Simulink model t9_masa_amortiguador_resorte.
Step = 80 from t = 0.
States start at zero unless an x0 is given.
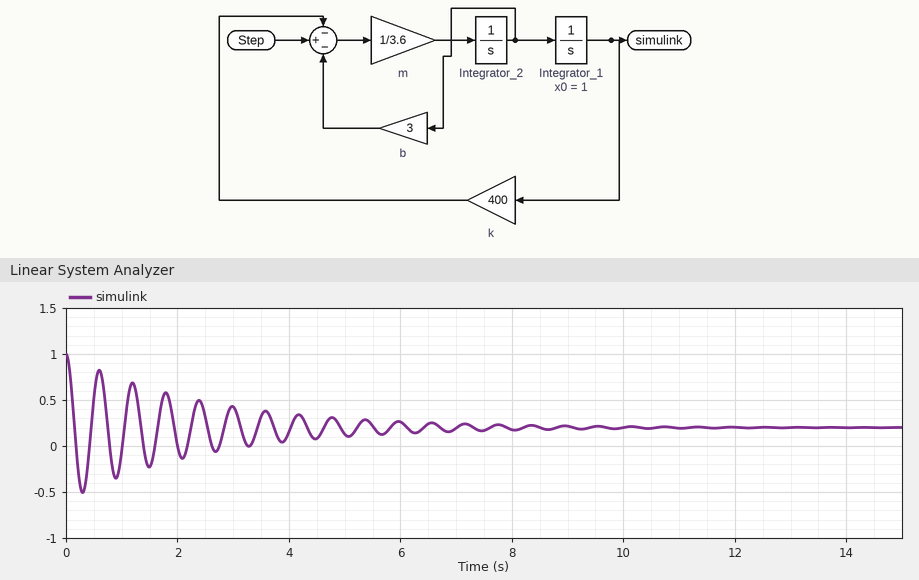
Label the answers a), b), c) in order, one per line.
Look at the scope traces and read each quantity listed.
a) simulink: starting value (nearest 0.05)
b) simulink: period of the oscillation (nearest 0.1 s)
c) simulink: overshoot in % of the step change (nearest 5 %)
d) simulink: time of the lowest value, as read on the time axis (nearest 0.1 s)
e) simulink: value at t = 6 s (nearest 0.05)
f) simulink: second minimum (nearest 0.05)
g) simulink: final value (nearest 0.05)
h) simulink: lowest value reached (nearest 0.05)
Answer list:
a) 1.00
b) 0.6 s
c) 90 %
d) 0.3 s
e) 0.25
f) -0.35
g) 0.20
h) -0.50
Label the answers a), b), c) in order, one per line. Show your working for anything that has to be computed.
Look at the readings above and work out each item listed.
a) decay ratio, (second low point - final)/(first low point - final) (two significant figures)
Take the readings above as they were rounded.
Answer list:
a) (-0.35 - 0.2) / (-0.5 - 0.2) = 0.79
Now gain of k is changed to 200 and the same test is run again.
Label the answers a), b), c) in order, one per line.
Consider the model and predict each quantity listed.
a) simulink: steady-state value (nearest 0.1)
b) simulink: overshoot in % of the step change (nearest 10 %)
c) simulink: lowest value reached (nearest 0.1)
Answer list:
a) 0.4
b) 80 %
c) -0.1
